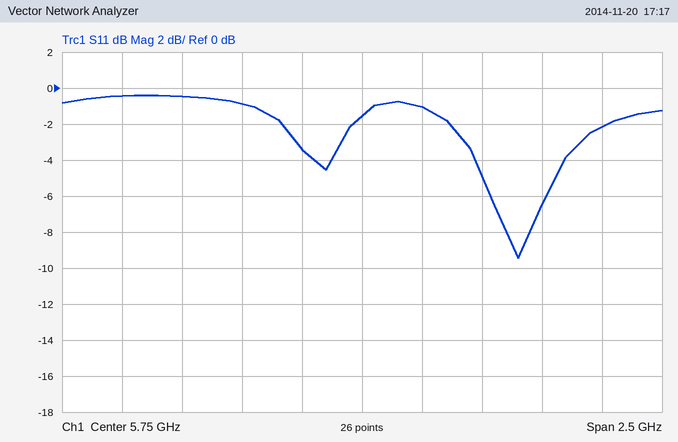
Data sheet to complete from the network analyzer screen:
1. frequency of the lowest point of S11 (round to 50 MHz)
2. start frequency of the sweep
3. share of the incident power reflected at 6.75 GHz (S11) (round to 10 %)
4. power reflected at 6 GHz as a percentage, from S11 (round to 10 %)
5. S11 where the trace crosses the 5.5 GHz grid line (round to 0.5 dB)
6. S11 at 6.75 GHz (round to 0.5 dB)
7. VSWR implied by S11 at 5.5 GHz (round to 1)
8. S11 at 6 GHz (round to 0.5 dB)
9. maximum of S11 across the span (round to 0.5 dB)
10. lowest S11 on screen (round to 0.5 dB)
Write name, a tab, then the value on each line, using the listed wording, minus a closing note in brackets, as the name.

frequency of the lowest point of S11	6.40 GHz
start frequency of the sweep	4.5 GHz
share of the incident power reflected at 6.75 GHz (S11)	60 %
power reflected at 6 GHz as a percentage, from S11	80 %
S11 where the trace crosses the 5.5 GHz grid line	-3.5 dB
S11 at 6.75 GHz	-2.0 dB
VSWR implied by S11 at 5.5 GHz	5
S11 at 6 GHz	-1.0 dB
maximum of S11 across the span	-0.5 dB
lowest S11 on screen	-9.5 dB
